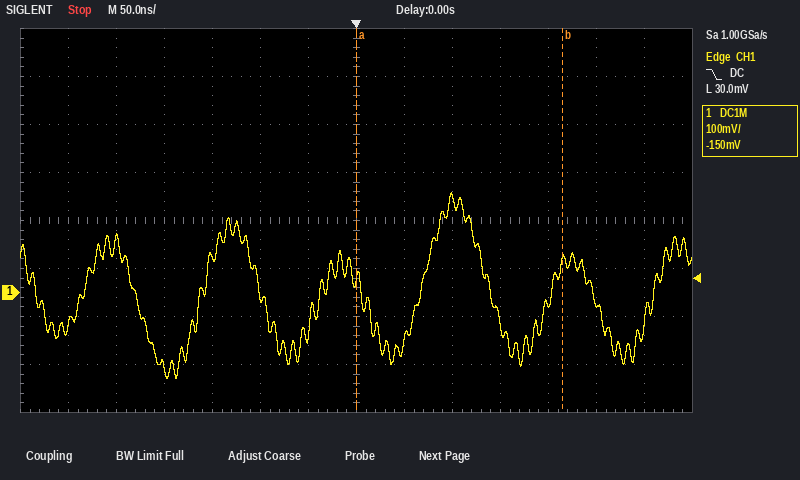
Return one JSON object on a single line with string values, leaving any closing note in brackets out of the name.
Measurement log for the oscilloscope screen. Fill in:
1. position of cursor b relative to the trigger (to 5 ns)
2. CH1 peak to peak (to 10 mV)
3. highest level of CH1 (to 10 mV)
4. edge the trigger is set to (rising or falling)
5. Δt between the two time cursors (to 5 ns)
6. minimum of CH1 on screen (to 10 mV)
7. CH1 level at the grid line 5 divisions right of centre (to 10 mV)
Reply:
{"position of cursor b relative to the trigger": "+215 ns", "CH1 peak to peak": "390 mV", "highest level of CH1": "210 mV", "edge the trigger is set to": "falling", "Δt between the two time cursors": "215 ns", "minimum of CH1 on screen": "-180 mV", "CH1 level at the grid line 5 divisions right of centre": "-20 mV"}
